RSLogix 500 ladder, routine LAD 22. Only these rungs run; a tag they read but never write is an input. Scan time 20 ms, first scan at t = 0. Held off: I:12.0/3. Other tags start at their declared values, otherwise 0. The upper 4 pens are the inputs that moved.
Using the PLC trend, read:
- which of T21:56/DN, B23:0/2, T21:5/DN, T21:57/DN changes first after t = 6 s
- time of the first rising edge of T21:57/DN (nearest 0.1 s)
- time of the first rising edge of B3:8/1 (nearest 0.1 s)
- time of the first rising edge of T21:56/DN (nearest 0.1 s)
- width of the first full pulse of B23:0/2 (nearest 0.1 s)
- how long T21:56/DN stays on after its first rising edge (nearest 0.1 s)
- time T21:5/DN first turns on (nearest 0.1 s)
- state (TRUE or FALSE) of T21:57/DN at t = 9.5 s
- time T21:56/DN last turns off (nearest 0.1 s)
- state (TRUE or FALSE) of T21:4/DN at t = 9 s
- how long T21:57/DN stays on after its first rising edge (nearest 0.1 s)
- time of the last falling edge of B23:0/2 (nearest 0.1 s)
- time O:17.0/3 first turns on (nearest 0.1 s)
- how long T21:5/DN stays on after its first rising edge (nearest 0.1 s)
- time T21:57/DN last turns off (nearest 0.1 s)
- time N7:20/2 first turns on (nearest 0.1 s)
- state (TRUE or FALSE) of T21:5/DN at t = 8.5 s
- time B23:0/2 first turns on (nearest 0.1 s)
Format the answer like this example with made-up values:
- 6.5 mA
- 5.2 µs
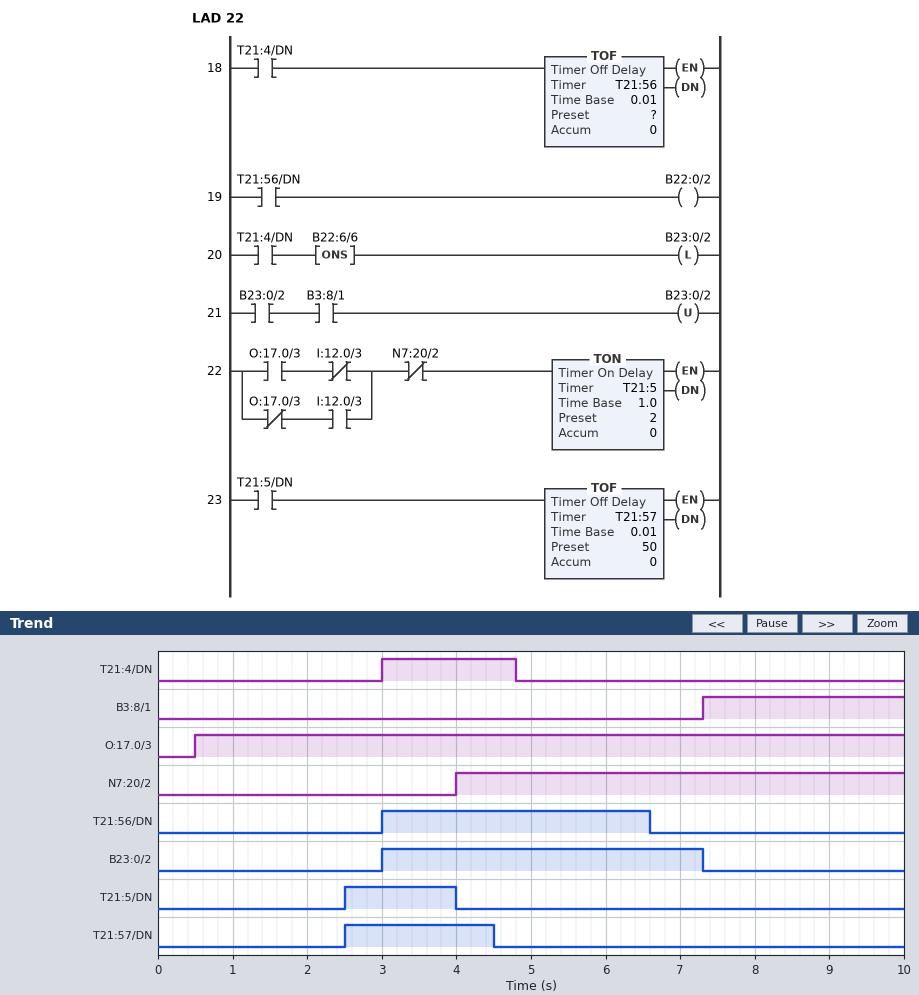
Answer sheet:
- T21:56/DN
- 2.5 s
- 7.3 s
- 3.0 s
- 4.3 s
- 3.6 s
- 2.5 s
- FALSE
- 6.6 s
- FALSE
- 2.0 s
- 7.3 s
- 0.5 s
- 1.5 s
- 4.5 s
- 4.0 s
- FALSE
- 3.0 s
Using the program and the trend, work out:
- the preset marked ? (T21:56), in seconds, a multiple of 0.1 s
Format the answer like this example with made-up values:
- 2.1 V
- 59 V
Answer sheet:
- 1.8 s
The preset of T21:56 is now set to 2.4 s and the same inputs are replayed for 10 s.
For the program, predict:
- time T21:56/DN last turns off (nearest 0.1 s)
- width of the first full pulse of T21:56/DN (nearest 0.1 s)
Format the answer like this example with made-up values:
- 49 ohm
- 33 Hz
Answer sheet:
- 7.2 s
- 4.2 s
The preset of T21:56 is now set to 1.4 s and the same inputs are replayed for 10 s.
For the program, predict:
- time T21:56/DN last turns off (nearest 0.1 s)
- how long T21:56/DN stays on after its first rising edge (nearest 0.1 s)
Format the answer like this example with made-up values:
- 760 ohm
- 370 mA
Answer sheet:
- 6.2 s
- 3.2 s
